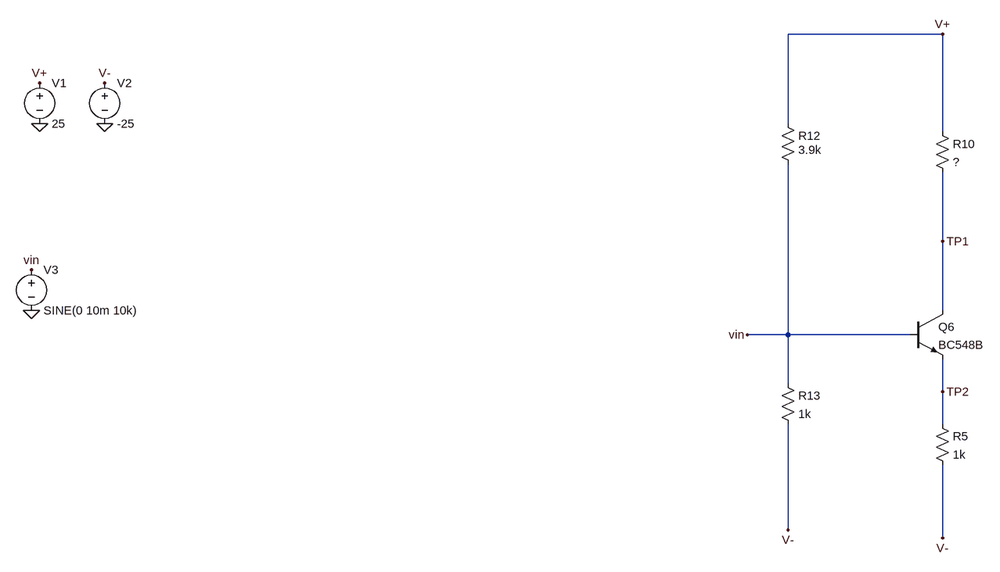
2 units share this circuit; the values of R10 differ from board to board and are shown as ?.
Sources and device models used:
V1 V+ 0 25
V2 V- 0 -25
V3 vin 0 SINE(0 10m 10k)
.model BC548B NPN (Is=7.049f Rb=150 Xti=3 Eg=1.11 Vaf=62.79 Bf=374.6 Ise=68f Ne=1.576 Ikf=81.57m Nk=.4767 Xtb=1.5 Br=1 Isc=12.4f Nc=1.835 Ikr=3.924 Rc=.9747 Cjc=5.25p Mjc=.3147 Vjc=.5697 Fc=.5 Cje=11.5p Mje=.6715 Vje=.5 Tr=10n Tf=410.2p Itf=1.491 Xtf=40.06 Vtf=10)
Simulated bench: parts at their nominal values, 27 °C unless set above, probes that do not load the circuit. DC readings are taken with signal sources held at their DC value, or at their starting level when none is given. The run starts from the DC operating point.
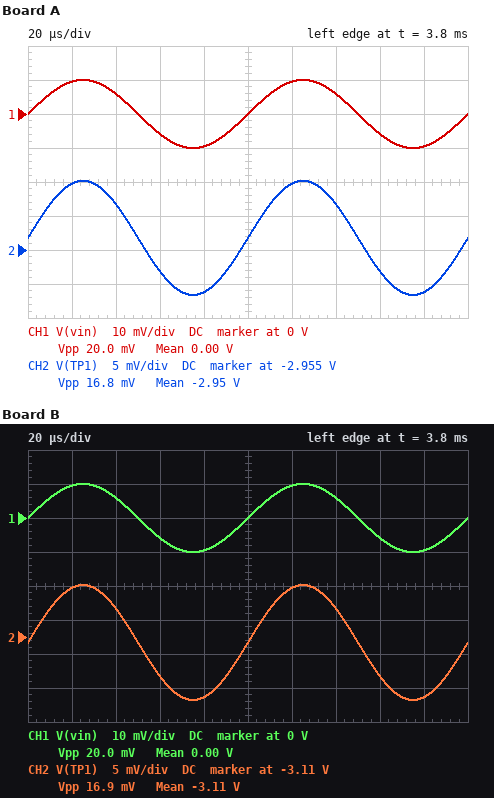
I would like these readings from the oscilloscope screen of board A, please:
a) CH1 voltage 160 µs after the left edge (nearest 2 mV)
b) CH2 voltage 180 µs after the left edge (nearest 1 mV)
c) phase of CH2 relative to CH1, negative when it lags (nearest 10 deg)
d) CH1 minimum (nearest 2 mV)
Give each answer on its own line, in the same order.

-6 mV
-2.961 V
0 deg
-10 mV
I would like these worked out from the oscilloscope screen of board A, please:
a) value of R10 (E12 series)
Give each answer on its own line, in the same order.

3.9 kΩ
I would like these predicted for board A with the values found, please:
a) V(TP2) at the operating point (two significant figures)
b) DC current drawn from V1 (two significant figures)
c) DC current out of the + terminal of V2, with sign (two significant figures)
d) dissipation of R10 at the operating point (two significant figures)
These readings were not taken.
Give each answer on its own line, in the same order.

-3.0 V
14 mA
-47 mA
200 mW
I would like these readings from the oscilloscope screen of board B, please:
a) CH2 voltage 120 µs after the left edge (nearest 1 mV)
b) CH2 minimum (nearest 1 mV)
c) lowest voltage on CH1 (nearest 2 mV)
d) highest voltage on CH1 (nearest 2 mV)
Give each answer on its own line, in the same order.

-3.103 V
-3.119 V
-10 mV
10 mV
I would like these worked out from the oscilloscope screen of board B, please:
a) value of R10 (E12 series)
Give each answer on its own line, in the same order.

4.7 kΩ
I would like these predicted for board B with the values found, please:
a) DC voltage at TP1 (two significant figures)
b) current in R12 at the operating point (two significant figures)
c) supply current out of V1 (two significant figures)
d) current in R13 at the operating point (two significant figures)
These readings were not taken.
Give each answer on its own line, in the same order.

-3.1 V
6.4 mA
12 mA
25 mA
